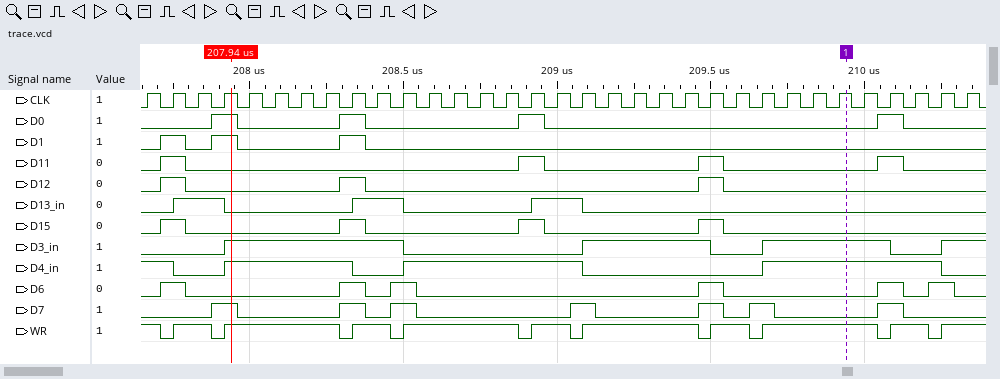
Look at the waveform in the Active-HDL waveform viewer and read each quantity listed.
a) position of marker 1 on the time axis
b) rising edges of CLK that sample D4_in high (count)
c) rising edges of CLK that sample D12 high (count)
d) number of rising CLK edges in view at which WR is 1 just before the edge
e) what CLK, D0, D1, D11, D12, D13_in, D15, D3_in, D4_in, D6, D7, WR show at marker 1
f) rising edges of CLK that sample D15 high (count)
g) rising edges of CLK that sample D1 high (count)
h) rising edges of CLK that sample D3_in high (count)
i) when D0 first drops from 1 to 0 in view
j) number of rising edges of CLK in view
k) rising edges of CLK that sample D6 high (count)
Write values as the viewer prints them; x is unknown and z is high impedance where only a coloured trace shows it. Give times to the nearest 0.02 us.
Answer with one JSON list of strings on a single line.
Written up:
["209.94 us", "21", "3", "23", "CLK=1, D0=0, D1=0, D11=0, D12=0, D13_in=0, D15=0, D3_in=1, D4_in=1, D6=0, D7=0, WR=1", "4", "3", "18", "207.96 us", "33", "6"]
